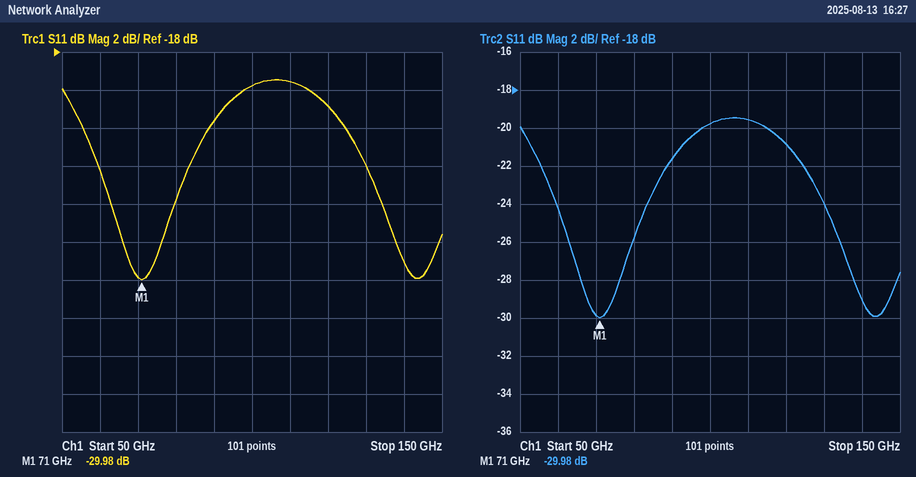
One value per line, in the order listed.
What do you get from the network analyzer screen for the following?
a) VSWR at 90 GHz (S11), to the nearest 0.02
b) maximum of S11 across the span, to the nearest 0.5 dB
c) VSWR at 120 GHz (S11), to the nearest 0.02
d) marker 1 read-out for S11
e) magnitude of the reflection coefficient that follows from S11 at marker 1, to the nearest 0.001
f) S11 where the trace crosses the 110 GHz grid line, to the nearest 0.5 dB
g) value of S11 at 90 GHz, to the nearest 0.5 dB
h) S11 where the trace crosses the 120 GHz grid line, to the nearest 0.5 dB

1.18
-19.5 dB
1.20
-29.98 dB
0.032
-19.5 dB
-21.5 dB
-21.0 dB
